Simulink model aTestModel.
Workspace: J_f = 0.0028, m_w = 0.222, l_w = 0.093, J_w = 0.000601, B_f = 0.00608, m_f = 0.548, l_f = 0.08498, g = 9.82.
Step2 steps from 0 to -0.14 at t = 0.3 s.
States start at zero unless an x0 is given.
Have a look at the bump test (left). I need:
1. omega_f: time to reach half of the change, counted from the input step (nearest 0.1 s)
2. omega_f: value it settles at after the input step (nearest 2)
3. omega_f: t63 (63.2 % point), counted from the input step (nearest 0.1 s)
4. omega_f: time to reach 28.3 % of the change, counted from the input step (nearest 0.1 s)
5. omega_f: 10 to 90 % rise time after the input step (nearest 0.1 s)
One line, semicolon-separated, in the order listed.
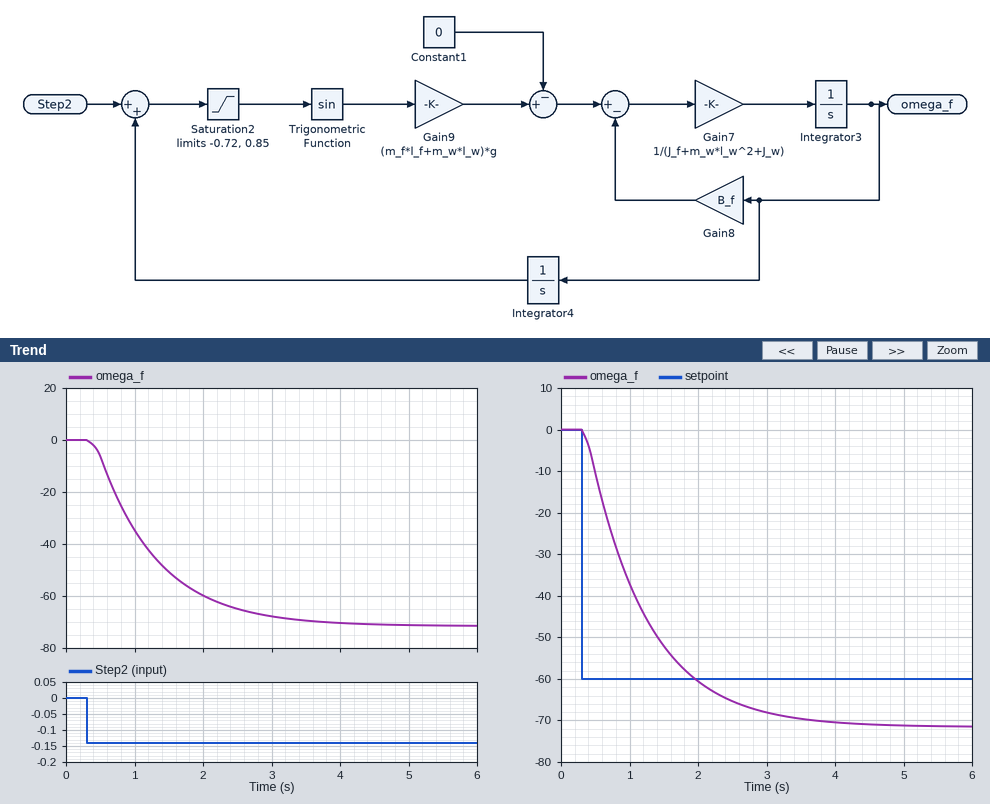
0.7 s; -72; 1.0 s; 0.4 s; 1.9 s
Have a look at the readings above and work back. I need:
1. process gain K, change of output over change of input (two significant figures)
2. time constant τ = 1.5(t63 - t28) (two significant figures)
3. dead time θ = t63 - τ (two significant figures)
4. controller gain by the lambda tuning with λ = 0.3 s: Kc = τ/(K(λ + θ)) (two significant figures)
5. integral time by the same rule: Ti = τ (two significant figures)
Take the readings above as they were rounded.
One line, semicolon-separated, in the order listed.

510; 0.90 s; 0.10 s; 0.0044; 0.90 s
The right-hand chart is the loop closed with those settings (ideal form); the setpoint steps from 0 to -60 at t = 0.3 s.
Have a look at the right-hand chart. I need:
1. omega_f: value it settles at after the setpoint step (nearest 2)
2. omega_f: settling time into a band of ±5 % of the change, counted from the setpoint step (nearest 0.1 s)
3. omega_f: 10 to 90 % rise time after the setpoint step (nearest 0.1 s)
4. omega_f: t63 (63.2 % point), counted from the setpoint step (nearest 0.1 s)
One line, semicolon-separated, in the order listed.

-72; 2.7 s; 1.9 s; 0.9 s
